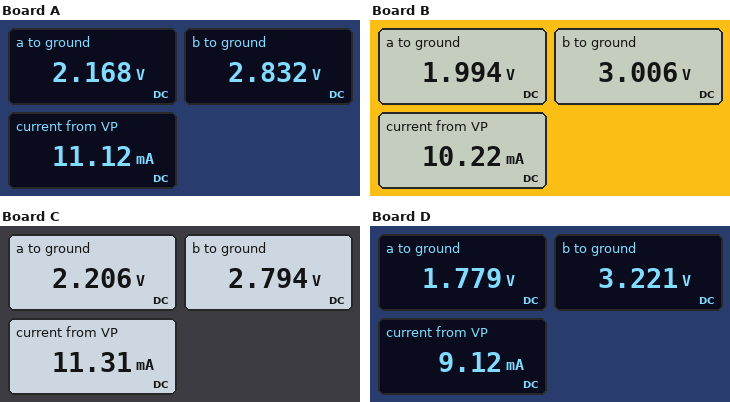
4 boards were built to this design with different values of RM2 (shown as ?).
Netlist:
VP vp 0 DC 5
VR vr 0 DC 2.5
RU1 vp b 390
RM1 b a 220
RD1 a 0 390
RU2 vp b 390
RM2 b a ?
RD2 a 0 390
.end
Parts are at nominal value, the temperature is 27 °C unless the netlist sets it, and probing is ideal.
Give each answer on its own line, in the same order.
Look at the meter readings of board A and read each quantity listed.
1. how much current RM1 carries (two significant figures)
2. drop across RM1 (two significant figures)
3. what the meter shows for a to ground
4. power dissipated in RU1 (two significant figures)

3.0 mA
660 mV
2.168 V
12 mW
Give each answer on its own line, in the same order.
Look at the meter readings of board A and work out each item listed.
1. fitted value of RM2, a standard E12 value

82 Ω
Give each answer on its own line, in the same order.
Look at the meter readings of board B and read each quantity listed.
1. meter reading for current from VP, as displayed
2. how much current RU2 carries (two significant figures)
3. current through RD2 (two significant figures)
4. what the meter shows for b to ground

10.22 mA
5.1 mA
5.1 mA
3.006 V
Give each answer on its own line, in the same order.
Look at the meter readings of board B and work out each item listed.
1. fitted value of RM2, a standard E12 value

180 Ω
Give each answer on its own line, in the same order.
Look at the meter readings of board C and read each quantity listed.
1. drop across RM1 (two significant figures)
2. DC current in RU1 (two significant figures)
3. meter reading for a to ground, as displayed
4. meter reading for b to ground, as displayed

590 mV
5.7 mA
2.206 V
2.794 V
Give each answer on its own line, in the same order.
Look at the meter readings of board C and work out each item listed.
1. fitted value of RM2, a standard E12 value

68 Ω
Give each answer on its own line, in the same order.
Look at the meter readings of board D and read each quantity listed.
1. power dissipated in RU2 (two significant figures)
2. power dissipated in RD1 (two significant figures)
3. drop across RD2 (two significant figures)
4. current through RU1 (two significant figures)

8.1 mW
8.1 mW
1.8 V
4.6 mA
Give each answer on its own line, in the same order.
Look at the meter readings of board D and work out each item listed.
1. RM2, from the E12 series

560 Ω
